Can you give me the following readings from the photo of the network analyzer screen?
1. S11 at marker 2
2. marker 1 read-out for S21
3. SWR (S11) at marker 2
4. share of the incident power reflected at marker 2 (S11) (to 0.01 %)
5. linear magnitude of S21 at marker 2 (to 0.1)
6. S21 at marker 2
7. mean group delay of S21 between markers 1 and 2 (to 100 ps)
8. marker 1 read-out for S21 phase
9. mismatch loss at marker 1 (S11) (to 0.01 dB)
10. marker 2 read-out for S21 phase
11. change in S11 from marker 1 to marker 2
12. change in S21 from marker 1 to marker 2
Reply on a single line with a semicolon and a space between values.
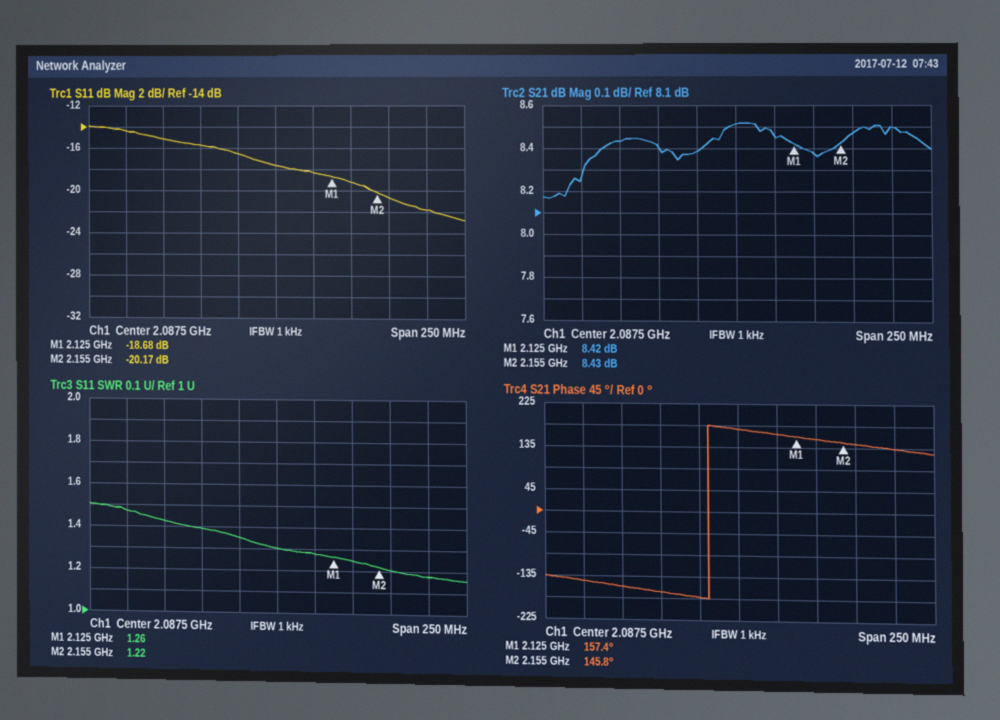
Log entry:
-20.17 dB; 8.42 dB; 1.22; 0.96 %; 2.6; 8.43 dB; 1.1 ns; 157.4°; 0.06 dB; 145.8°; -1.49 dB; 0.01 dB
